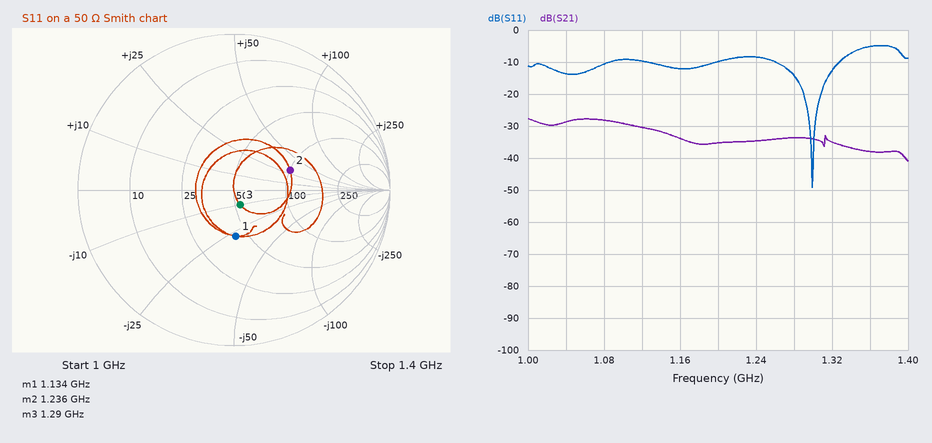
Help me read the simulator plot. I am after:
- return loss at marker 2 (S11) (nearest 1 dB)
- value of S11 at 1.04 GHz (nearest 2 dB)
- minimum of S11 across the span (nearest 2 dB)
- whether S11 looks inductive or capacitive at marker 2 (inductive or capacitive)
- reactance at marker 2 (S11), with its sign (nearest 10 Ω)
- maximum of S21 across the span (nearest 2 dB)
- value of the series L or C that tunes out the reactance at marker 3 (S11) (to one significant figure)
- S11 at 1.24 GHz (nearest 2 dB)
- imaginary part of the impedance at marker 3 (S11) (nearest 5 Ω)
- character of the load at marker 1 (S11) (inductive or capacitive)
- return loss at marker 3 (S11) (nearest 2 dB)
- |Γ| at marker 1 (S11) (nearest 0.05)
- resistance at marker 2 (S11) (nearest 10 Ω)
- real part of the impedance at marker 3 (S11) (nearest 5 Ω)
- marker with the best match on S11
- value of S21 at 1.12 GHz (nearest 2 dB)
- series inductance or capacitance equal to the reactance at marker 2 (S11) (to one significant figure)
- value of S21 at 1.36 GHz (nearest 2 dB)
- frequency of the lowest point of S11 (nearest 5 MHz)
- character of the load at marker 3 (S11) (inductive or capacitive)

8 dB
-14 dB
-50 dB
inductive
+30 Ω
-28 dB
1 nH
-8 dB
-10 Ω
capacitive
20 dB
0.30
100 Ω
55 Ω
marker 3
-30 dB
4 nH
-38 dB
1.300 GHz
capacitive
